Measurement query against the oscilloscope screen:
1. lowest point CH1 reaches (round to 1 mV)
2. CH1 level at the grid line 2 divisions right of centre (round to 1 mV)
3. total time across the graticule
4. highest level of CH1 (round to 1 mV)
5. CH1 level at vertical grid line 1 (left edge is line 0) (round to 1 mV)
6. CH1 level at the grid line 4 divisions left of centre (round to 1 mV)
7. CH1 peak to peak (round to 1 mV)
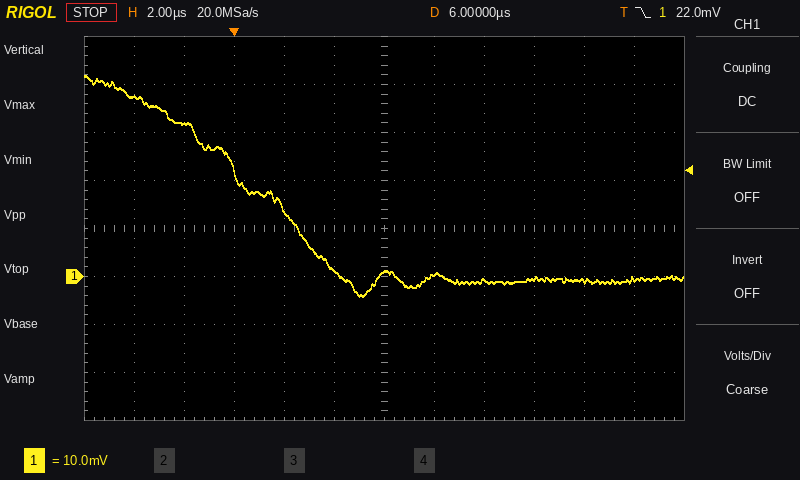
-4 mV
-1 mV
24 µs
42 mV
37 mV
32 mV
46 mV
